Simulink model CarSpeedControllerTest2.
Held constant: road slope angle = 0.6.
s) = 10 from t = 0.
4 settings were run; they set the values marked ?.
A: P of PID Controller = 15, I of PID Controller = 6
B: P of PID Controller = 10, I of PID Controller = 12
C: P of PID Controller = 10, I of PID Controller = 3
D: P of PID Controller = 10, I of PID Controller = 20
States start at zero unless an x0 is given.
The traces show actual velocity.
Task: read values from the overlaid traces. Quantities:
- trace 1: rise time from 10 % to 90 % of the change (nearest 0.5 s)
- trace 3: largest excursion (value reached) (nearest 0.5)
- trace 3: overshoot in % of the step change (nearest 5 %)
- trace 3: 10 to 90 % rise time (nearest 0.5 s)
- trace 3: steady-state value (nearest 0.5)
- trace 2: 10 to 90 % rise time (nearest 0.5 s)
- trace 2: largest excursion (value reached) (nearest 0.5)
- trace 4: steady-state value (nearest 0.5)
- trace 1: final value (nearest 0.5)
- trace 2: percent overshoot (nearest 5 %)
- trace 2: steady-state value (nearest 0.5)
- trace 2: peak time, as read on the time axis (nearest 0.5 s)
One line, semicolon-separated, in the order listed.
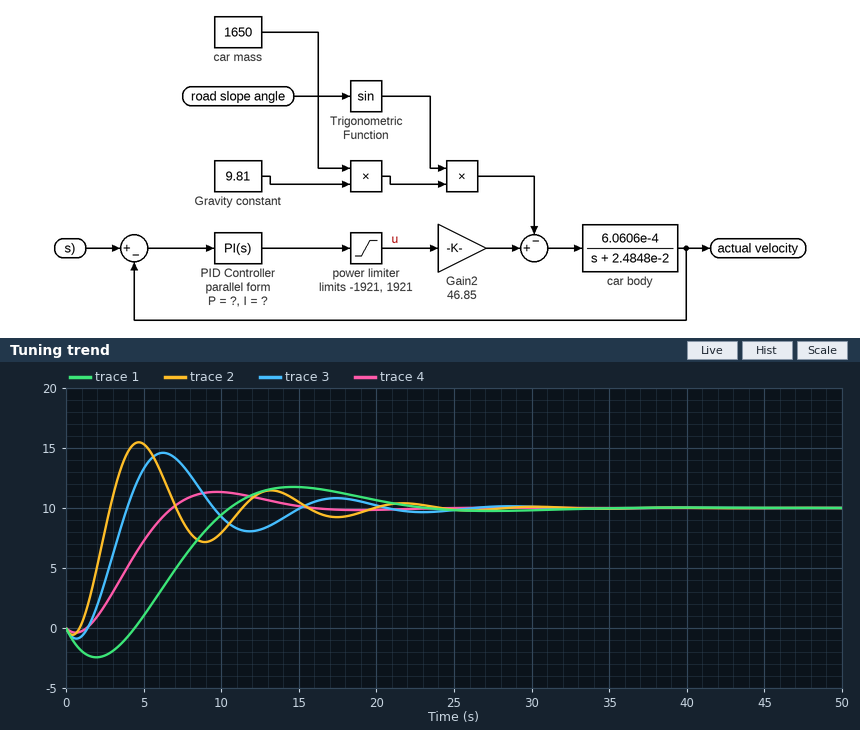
4.5 s; 14.5; 45 %; 2.0 s; 10.0; 1.5 s; 15.5; 10.0; 10.0; 55 %; 10.0; 4.5 s
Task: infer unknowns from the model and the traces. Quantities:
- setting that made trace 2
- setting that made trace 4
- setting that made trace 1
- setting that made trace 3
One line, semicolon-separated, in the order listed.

D; A; C; B
